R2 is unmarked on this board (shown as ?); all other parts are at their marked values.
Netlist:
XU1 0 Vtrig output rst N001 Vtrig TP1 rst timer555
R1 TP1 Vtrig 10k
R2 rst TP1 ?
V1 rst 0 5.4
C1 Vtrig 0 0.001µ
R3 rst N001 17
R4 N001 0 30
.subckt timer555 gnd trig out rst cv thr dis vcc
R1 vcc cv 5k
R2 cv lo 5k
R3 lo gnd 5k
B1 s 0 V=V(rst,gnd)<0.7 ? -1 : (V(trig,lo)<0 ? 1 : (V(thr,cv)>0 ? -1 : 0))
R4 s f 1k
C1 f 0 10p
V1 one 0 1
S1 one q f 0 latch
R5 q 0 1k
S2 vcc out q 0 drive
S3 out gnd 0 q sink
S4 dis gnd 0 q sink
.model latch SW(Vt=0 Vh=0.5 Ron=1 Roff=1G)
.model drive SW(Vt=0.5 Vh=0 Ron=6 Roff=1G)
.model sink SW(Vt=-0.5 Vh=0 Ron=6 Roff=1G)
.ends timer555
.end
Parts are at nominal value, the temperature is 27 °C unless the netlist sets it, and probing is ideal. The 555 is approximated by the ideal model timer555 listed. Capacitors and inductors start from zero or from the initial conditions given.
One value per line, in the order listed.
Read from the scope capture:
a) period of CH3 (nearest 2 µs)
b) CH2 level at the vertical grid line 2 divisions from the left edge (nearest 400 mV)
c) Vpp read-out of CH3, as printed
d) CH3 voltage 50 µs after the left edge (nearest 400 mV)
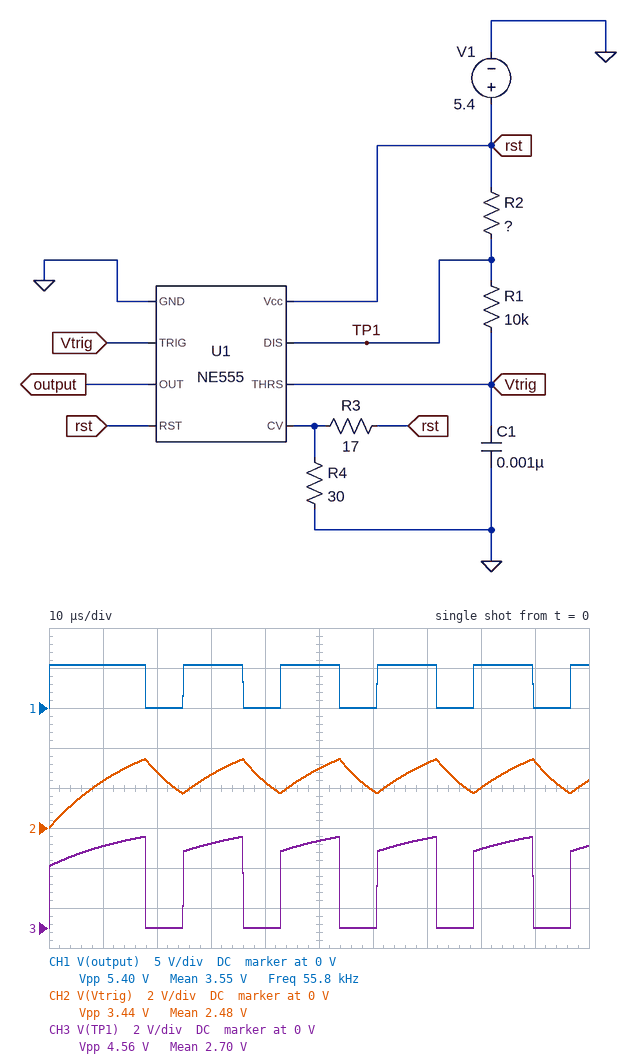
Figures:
18 µs
2.8 V
4.56 V
4.4 V
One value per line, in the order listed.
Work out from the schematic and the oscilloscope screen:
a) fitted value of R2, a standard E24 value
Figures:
7.5 kΩ
